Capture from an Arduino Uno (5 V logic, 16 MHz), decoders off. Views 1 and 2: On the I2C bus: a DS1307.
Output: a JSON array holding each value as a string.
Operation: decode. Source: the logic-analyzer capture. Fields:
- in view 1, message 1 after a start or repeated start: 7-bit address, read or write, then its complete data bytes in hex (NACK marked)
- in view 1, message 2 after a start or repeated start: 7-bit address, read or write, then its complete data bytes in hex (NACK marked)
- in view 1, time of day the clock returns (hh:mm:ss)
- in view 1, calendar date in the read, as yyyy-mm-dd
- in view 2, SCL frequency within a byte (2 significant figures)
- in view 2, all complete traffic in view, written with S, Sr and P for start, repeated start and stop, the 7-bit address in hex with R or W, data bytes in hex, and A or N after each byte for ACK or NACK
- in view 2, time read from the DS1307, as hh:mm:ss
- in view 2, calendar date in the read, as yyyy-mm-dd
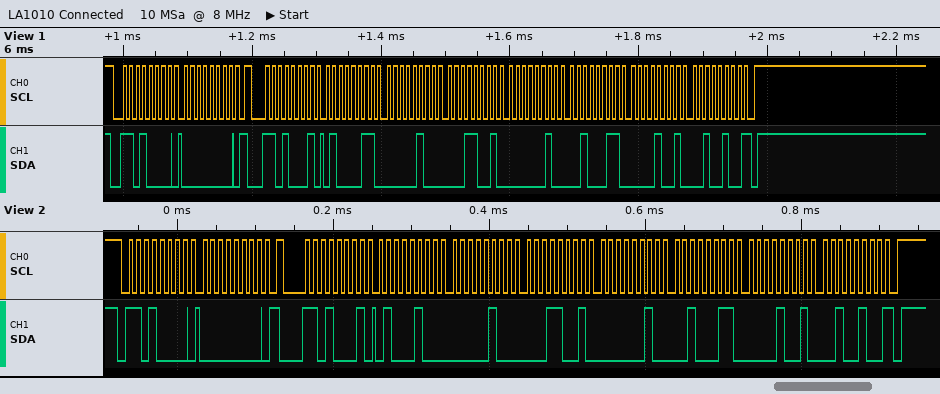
["0x68 write: 00", "0x68 read: 43 04 19 02 23 09 24 NACK", "19:04:43", "2024-09-23", "100 kHz", "S 68W A 00 A Sr 68R A 44 A 04 A 19 A 02 A 23 A 09 A 24 N P", "19:04:44", "2024-09-23"]
